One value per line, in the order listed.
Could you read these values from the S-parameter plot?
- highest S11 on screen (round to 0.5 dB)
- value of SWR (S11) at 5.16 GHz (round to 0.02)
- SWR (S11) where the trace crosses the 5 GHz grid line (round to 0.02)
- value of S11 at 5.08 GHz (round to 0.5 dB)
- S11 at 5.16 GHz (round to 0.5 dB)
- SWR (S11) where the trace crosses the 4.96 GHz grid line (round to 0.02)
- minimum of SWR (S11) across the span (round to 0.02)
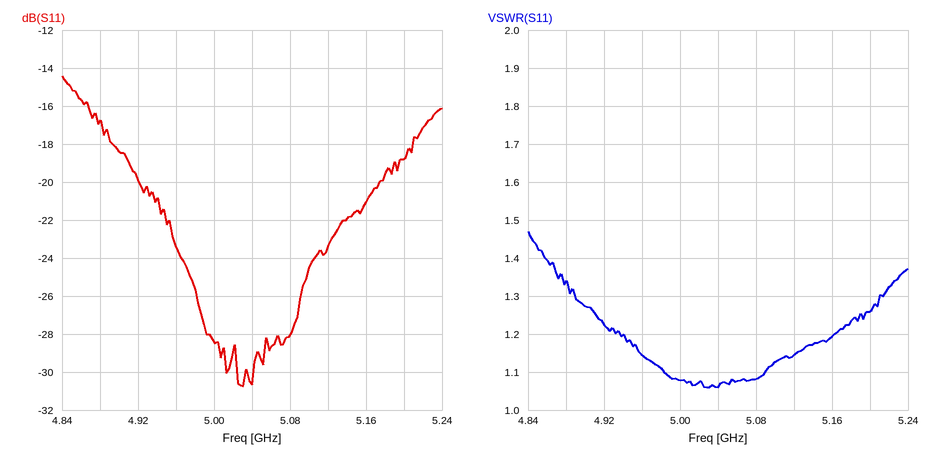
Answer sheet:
-14.5 dB
1.20
1.08
-28.0 dB
-21.0 dB
1.14
1.06
